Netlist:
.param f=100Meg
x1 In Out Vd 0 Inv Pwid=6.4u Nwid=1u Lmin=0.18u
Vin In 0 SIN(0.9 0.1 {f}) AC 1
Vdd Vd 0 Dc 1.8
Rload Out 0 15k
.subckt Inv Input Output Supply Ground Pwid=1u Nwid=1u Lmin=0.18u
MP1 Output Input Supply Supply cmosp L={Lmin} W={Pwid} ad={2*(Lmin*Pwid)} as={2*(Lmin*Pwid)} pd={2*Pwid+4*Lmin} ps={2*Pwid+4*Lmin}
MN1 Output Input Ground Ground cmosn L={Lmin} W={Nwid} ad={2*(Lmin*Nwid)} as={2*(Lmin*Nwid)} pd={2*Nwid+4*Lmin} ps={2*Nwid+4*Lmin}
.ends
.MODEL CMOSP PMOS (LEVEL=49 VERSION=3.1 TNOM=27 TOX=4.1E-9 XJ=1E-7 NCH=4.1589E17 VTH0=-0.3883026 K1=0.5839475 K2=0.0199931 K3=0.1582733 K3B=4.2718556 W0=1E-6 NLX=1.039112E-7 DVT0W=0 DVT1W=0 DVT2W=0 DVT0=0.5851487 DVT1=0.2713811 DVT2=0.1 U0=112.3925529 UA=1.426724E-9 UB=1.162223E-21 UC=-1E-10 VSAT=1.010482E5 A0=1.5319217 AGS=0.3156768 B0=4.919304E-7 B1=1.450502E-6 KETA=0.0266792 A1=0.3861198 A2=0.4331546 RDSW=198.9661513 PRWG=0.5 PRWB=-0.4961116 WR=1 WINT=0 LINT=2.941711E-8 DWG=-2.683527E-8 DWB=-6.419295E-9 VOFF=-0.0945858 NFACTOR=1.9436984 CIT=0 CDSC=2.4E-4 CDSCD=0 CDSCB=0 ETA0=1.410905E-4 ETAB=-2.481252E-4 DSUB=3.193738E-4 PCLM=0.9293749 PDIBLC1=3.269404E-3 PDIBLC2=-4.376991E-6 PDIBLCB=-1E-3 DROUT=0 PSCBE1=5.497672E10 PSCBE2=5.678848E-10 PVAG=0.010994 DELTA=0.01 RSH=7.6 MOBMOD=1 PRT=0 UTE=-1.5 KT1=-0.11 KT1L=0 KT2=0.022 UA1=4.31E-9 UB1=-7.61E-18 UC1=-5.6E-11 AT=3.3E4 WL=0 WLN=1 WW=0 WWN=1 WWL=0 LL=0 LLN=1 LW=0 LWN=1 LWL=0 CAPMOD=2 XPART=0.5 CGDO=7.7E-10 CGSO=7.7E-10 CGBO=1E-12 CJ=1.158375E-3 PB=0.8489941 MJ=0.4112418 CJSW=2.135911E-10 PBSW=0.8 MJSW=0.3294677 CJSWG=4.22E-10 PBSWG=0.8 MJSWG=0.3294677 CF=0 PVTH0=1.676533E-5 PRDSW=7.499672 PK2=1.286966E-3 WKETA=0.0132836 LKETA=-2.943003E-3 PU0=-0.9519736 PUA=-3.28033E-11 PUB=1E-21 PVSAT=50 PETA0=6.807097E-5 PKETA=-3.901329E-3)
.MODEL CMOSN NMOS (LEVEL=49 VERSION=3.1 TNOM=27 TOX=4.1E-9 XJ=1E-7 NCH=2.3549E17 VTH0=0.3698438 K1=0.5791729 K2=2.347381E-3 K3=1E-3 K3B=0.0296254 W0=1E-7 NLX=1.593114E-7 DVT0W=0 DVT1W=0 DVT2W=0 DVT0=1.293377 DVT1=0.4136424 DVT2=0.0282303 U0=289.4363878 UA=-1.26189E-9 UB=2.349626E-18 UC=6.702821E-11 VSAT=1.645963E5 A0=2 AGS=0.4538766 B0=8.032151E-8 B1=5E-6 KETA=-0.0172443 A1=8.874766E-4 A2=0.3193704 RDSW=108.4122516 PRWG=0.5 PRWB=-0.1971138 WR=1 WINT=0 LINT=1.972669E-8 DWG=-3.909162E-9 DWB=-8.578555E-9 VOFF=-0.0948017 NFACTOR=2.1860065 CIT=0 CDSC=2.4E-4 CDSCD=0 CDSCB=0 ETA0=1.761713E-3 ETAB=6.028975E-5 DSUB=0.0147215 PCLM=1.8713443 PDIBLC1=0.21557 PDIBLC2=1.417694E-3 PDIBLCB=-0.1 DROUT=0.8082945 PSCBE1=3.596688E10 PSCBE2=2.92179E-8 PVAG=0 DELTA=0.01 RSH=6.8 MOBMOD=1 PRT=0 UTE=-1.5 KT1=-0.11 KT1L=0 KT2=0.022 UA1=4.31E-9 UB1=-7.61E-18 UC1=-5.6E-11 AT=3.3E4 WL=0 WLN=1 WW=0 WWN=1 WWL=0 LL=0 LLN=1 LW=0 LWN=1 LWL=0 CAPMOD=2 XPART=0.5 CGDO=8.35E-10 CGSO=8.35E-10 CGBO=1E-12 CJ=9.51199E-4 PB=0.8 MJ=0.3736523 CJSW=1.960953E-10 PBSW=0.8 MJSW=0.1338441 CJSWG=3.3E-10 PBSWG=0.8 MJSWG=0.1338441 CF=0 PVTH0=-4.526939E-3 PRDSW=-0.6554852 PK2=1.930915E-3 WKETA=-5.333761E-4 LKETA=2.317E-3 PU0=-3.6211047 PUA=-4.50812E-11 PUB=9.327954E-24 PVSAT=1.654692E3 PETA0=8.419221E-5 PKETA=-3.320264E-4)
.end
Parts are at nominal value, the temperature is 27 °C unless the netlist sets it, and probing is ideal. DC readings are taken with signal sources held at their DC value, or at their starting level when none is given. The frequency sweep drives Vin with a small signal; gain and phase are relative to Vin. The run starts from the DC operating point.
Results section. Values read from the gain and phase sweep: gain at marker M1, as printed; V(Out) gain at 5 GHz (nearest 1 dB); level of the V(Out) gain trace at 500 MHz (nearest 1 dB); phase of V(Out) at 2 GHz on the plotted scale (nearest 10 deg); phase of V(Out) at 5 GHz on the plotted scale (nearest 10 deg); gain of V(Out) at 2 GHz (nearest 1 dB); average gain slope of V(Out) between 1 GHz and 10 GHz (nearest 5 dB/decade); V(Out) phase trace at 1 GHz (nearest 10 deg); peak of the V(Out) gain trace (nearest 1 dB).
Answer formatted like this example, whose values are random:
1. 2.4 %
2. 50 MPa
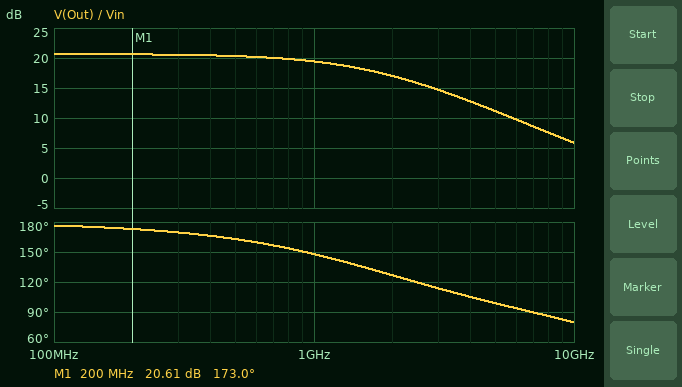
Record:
1. 20.61 dB
2. 11 dB
3. 20 dB
4. 130 deg
5. 100 deg
6. 17 dB
7. -15 dB/decade
8. 150 deg
9. 21 dB
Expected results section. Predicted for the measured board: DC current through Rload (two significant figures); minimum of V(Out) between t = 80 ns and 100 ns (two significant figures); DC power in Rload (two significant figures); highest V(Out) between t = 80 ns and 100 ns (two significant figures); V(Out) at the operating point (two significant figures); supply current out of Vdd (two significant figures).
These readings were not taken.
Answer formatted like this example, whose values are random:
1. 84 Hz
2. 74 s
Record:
1. 77 µA
2. 220 mV
3. 89 µW
4. 1.6 V
5. 1.2 V
6. 240 µA
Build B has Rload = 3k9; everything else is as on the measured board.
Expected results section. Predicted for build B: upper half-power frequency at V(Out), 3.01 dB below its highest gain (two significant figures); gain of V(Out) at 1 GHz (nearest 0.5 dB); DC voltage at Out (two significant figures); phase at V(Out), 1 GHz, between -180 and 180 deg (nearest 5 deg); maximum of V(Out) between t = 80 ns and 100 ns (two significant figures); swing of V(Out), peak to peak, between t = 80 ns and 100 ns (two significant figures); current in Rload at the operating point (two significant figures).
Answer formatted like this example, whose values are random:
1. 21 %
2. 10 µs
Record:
1. 4.6 GHz
2. 13.0 dB
3. 450 mV
4. 165 deg
5. 940 mV
6. 780 mV
7. 120 µA
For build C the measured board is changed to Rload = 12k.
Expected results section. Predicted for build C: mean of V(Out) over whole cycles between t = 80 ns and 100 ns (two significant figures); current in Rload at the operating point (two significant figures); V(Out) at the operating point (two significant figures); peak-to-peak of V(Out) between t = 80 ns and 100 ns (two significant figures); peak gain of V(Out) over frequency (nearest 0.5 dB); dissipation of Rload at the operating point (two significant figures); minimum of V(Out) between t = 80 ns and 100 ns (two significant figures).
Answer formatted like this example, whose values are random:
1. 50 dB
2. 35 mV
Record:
1. 940 mV
2. 85 µA
3. 1.0 V
4. 1.3 V
5. 20.5 dB
6. 87 µW
7. 210 mV
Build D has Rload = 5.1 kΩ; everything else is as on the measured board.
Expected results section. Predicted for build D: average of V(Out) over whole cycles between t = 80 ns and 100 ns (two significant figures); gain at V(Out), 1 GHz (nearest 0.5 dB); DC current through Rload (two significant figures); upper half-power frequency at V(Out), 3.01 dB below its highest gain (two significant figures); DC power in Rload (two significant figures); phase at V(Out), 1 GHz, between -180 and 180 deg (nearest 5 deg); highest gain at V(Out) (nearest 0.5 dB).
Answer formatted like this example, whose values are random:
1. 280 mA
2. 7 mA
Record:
1. 610 mV
2. 15.0 dB
3. 110 µA
4. 3.5 GHz
5. 61 µW
6. 160 deg
7. 15.5 dB
